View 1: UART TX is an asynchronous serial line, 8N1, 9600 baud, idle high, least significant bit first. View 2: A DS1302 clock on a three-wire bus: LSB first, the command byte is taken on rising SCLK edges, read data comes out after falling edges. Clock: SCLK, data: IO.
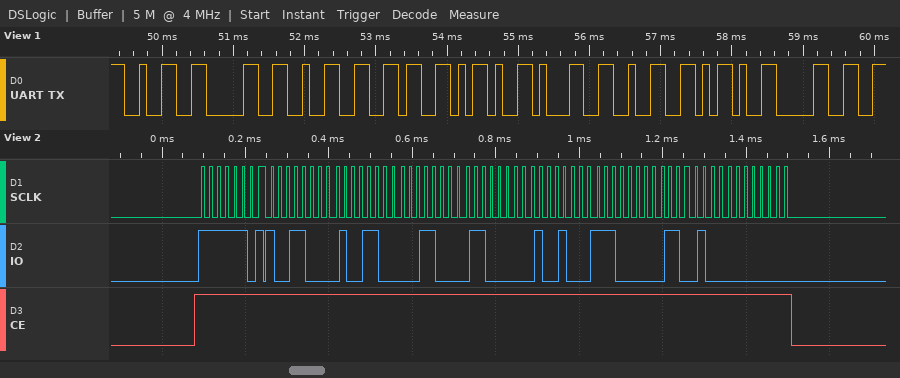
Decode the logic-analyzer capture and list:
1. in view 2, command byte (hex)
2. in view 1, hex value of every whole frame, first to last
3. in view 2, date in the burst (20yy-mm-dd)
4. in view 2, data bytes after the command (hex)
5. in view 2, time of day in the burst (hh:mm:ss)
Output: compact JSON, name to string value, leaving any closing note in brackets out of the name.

{"in view 2, command byte": "0xBF", "in view 1, hex value of every whole frame, first to last": "32 30 32 36 2D 31 32 2D 30", "in view 2, date in the burst": "2026-12-06", "in view 2, data bytes after the command": "19 32 18 06 12 07 26 00", "in view 2, time of day in the burst": "18:32:19"}
